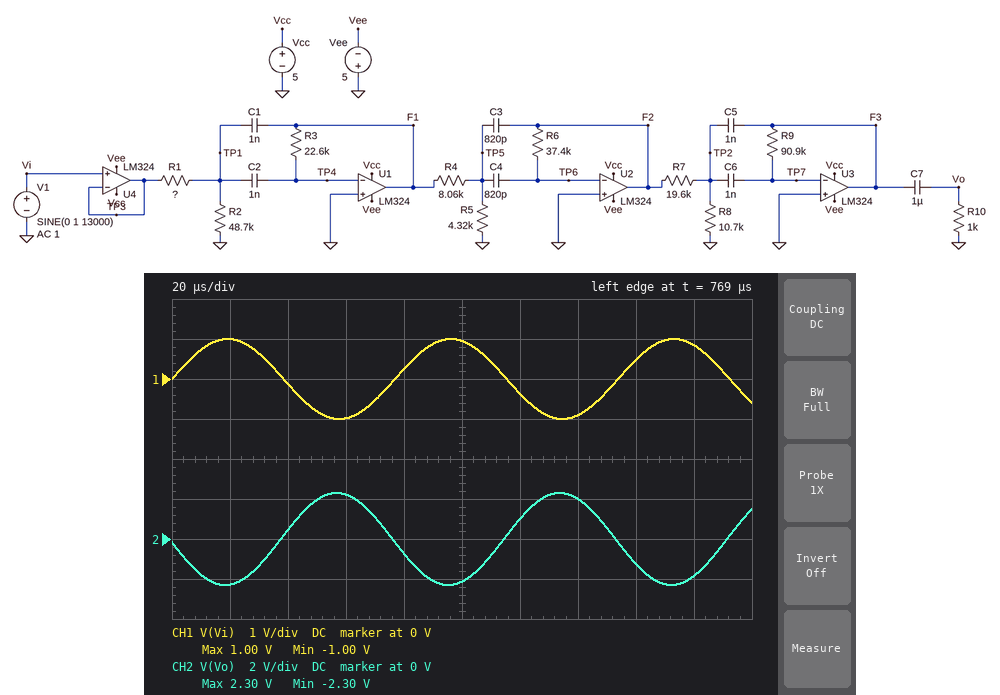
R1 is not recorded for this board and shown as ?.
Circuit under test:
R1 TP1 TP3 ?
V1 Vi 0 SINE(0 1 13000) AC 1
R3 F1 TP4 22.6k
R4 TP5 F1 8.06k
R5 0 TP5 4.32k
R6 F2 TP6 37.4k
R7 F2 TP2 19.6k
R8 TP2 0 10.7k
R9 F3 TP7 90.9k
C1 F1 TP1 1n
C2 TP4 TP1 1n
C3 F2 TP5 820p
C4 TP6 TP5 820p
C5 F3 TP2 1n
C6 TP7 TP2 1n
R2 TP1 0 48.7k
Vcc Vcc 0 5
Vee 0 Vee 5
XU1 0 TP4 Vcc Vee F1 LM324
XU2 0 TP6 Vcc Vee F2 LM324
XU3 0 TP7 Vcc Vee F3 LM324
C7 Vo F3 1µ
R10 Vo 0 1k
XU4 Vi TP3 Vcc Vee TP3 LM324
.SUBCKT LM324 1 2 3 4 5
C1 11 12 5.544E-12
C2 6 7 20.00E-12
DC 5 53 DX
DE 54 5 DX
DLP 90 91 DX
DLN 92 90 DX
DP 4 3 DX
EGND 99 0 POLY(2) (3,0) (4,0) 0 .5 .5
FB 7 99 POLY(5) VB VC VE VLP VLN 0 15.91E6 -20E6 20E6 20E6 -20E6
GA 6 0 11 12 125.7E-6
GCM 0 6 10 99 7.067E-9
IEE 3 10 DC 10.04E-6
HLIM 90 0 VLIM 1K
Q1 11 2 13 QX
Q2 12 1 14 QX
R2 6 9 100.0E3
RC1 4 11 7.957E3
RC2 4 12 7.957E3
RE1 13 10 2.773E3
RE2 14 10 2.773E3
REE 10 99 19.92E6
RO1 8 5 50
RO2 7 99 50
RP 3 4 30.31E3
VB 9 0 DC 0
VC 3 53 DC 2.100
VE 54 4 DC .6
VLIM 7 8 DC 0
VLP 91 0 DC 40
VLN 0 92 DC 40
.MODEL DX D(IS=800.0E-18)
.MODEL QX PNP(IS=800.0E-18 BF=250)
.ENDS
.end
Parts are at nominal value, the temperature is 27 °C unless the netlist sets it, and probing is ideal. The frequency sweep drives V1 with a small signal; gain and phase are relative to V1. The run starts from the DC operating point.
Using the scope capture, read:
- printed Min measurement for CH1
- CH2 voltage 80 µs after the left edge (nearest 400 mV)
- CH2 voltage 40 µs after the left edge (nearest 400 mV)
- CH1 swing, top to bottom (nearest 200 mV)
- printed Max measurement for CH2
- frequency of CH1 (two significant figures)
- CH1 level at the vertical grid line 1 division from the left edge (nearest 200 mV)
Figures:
-1.00 V
-800 mV
400 mV
2.0 V
2.30 V
13 kHz
1.0 V
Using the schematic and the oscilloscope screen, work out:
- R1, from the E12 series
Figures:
4.7 kΩ
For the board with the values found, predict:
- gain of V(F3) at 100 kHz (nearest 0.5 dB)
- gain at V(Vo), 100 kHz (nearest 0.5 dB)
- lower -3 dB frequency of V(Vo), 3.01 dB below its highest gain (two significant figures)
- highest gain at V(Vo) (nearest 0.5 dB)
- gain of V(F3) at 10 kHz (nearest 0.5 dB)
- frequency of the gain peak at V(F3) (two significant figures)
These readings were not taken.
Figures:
-44.0 dB
-44.0 dB
12 kHz
9.0 dB
4.0 dB
16 kHz
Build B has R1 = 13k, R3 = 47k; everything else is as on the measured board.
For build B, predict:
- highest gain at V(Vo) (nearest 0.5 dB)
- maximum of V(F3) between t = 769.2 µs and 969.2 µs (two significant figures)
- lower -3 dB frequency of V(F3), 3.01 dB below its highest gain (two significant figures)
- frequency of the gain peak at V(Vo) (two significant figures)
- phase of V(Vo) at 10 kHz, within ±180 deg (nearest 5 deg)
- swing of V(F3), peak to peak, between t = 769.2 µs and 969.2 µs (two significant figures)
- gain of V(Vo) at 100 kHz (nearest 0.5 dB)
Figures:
6.5 dB
1.1 V
5.7 kHz
7.1 kHz
150 deg
2.3 V
-53.0 dB
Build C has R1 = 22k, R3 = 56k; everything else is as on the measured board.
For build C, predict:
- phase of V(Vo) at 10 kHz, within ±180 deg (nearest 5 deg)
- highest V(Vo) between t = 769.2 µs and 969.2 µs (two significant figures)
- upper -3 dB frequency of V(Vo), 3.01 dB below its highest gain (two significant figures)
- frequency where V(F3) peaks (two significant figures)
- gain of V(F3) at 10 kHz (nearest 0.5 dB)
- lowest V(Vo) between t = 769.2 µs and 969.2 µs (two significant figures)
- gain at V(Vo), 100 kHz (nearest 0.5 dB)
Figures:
135 deg
620 mV
8.8 kHz
6.6 kHz
-2.0 dB
-620 mV
-57.5 dB
